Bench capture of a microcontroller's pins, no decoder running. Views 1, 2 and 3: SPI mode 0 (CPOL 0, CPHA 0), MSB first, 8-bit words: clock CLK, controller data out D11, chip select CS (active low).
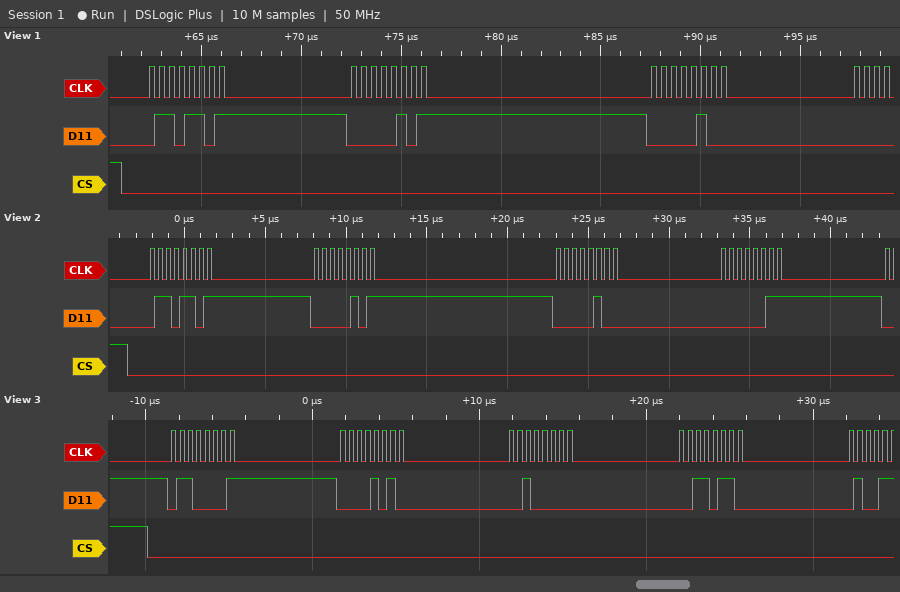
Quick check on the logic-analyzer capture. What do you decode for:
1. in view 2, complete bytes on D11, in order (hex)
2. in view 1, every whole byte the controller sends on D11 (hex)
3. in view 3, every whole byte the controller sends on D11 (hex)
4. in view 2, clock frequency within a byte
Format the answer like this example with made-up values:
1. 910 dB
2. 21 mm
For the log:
1. 6D 05 04 03
2. 6D 05 04
3. 0x61 0x0A 0x20 0x36
4. 2 MHz
